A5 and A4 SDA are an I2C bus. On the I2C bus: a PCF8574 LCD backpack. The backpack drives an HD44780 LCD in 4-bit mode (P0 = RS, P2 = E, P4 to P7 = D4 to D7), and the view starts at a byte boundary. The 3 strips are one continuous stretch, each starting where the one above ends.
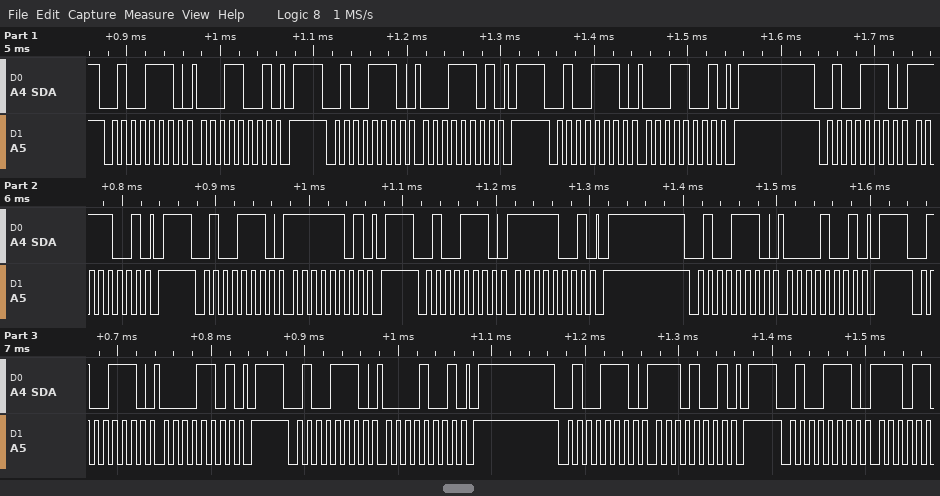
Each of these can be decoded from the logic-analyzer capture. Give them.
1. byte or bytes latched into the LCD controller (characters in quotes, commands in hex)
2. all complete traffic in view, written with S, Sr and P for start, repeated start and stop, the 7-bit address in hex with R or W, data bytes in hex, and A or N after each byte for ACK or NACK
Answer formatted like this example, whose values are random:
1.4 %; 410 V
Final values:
data 0x1F; S 27W A 19 A P S 27W A 1D A P S 27W A 19 A P S 27W A F9 A P S 27W A FD A P S 27W A F9 A P S 27W A 09 A P S 27W A 0D A P S 27W A 09 A P S 27W A E9 A P S 27W A
